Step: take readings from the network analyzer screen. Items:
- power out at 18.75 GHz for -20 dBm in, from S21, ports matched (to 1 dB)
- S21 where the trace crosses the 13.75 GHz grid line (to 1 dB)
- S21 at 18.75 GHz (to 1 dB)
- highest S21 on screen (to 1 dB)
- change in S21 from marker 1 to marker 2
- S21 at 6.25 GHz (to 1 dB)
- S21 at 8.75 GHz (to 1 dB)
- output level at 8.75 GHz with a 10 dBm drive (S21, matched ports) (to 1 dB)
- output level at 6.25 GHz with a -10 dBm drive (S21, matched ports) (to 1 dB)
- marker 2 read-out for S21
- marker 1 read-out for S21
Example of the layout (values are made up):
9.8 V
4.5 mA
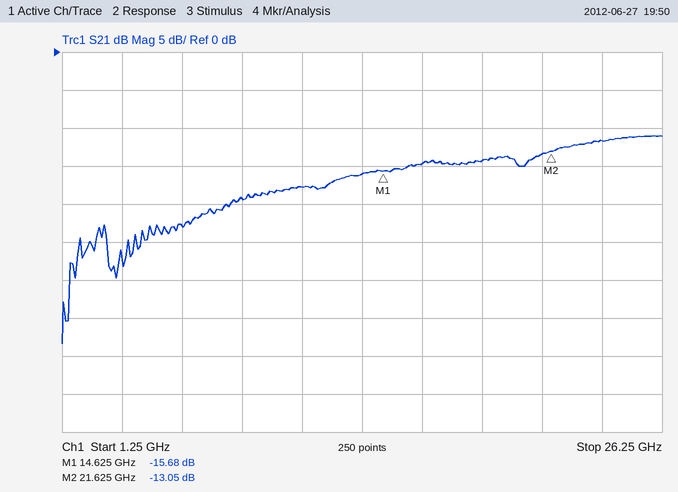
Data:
-34 dBm
-16 dB
-14 dB
-11 dB
2.63 dB
-23 dB
-19 dB
-9 dBm
-33 dBm
-13.05 dB
-15.68 dB
